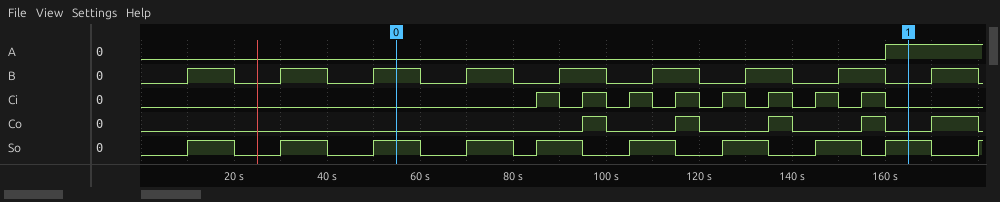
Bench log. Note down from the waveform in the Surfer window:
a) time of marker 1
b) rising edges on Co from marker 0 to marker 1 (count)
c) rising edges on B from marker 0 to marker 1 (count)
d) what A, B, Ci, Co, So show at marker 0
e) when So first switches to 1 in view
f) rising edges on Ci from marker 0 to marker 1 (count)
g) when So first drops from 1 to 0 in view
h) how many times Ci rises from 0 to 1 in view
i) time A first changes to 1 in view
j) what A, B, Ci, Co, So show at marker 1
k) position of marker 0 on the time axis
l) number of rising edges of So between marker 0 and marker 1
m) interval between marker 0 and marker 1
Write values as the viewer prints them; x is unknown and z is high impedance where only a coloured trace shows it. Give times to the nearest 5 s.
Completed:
165 s
4
5
A=0, B=1, Ci=0, Co=0, So=1
10 s
8
20 s
8
160 s
A=1, B=0, Ci=0, Co=0, So=1
55 s
6
110 s
